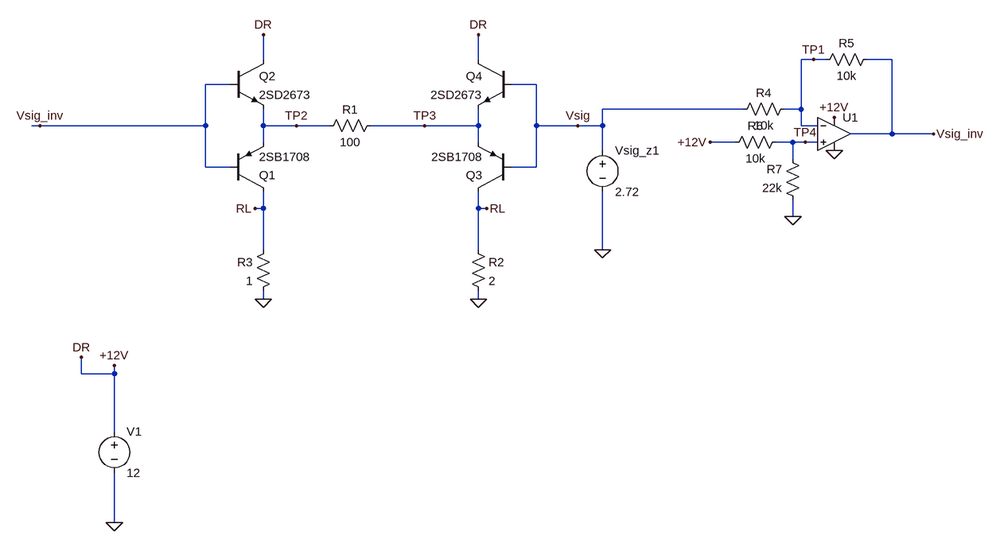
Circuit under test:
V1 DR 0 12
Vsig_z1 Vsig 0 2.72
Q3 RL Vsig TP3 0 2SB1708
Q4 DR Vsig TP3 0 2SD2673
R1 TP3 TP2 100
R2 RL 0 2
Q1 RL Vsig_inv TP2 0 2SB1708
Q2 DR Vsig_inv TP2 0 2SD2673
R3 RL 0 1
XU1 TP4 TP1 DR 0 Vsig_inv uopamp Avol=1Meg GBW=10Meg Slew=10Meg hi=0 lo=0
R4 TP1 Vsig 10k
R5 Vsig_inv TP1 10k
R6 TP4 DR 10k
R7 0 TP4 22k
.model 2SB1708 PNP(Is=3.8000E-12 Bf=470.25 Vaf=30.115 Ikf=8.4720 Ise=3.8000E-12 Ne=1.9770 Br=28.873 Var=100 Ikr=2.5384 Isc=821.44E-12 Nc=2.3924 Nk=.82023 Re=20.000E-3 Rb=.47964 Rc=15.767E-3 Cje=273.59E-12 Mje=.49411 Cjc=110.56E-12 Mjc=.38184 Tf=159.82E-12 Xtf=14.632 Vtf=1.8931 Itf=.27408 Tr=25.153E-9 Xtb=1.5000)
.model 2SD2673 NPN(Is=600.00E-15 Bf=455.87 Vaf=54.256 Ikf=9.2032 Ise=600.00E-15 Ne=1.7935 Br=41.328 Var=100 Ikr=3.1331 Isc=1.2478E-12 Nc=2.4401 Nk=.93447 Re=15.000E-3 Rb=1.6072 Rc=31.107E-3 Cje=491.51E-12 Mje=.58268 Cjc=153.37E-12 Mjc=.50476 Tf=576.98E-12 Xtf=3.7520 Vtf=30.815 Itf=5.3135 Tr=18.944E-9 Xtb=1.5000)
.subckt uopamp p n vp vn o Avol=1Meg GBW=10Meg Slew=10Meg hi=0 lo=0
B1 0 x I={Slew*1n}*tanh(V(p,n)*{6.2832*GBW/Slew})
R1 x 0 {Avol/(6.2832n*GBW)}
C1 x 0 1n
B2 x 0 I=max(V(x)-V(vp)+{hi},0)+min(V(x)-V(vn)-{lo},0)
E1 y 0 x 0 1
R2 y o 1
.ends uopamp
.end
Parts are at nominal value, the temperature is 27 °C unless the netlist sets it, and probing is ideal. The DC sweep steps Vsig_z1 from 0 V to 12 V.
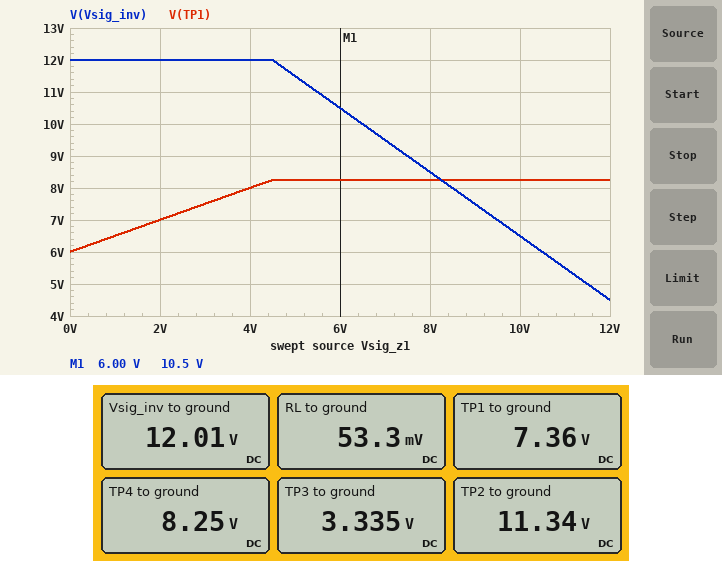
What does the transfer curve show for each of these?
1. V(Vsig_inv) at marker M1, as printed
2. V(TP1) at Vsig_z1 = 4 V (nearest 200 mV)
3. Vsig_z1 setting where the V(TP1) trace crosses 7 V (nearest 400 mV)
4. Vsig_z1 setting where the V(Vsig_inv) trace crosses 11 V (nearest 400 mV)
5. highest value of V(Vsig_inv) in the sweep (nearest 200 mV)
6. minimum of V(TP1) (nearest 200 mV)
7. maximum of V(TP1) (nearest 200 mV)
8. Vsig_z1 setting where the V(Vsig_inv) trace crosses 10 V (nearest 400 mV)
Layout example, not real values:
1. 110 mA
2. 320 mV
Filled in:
1. 10.5 V
2. 8.0 V
3. 2.0 V
4. 5.6 V
5. 12.0 V
6. 6.0 V
7. 8.2 V
8. 6.4 V
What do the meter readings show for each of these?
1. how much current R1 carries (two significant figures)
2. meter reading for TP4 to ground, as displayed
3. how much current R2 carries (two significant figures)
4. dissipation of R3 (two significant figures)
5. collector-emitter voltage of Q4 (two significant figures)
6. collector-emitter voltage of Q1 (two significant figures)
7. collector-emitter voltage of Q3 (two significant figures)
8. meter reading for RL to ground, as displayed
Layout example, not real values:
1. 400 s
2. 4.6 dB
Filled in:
1. 80 mA
2. 8.25 V
3. 27 mA
4. 2.8 mW
5. 8.7 V
6. -11 V
7. -3.3 V
8. 53.3 mV
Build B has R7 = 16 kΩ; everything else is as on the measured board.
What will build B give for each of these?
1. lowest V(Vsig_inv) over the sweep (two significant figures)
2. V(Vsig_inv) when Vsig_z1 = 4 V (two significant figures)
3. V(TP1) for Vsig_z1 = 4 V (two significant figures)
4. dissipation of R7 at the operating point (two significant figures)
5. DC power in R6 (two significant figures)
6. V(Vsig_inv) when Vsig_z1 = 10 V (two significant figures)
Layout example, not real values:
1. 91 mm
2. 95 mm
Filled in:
1. 2.8 V
2. 11 V
3. 7.4 V
4. 3.4 mW
5. 2.1 mW
6. 4.8 V
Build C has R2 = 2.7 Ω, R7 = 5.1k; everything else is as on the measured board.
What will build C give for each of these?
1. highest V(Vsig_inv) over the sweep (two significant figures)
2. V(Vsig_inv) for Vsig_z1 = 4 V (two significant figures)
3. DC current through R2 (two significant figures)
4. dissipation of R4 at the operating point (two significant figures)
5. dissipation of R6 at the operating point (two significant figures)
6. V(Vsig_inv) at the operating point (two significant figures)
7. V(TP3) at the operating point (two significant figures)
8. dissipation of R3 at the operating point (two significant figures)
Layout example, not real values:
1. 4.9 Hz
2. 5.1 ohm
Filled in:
1. 8.1 V
2. 4.1 V
3. 4.0 mA
4. 180 µW
5. 6.3 mW
6. 5.4 V
7. 3.3 V
8. 120 µW
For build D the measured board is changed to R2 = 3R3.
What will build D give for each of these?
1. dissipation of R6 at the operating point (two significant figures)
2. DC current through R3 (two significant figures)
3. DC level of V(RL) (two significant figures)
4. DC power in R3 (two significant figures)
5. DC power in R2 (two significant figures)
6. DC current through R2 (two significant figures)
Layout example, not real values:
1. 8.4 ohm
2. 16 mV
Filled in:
1. 1.4 mW
2. 61 mA
3. 61 mV
4. 3.8 mW
5. 1.1 mW
6. 19 mA
